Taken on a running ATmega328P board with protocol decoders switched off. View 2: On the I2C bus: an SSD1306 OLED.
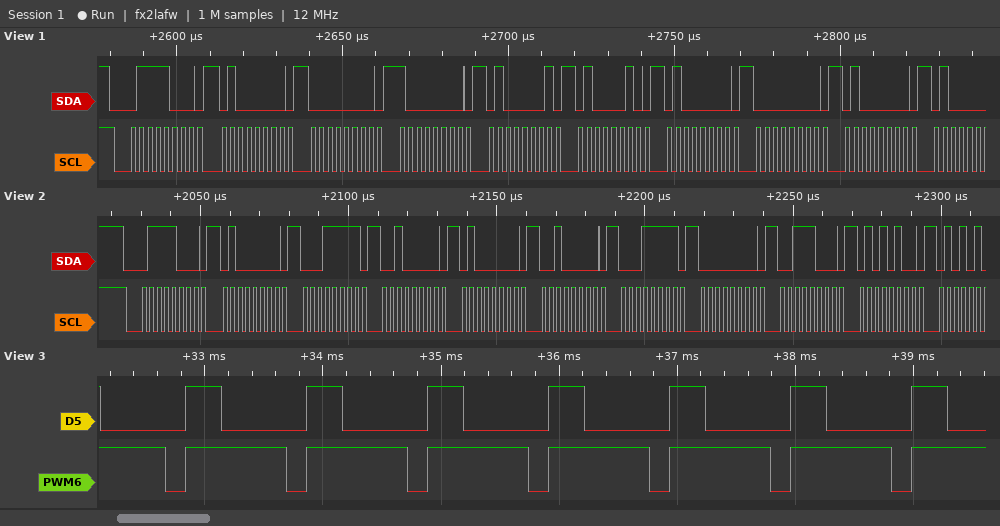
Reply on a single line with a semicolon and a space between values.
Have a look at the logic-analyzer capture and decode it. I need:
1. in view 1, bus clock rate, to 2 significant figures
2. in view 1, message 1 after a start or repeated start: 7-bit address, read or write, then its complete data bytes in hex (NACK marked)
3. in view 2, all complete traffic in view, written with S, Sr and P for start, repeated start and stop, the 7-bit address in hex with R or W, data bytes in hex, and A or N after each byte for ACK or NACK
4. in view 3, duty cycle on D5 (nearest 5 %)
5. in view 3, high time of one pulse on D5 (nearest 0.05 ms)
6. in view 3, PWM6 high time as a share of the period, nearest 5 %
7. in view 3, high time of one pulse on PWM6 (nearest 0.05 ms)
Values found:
400 kHz; 0x3C write: 40 00 80 41 42 40 00 40; S 3CW A 40 A 1F A 20 A 40 A 20 A 1F A 00 A 38 A 54 A; 30 %; 0.30 ms; 85 %; 0.85 ms
